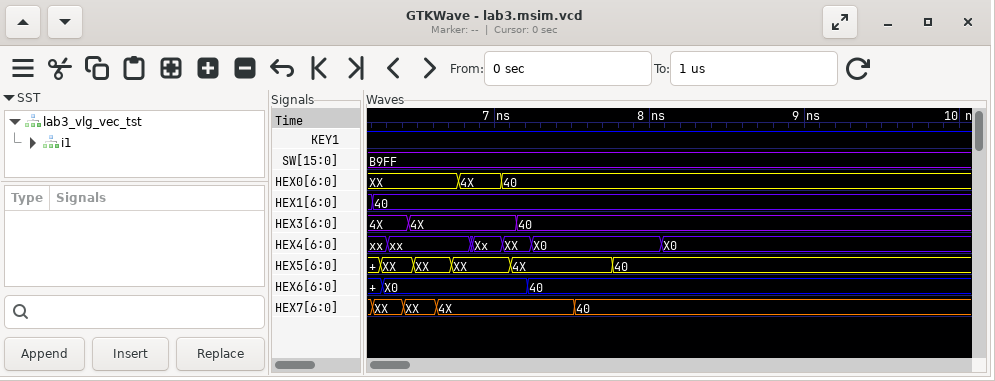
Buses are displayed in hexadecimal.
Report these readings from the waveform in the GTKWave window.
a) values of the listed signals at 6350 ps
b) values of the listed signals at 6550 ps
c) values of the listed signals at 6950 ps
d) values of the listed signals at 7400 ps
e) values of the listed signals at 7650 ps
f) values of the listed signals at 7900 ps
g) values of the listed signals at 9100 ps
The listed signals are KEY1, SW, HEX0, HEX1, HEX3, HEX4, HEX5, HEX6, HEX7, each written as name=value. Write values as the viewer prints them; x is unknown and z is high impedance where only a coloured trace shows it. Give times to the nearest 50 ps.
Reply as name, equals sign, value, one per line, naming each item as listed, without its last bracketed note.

values of the listed signals at 6350 ps = KEY1=1, SW=B9FF, HEX0=XX, HEX1=40, HEX3=4X, HEX4=xx, HEX5=XX, HEX6=X0, HEX7=XX
values of the listed signals at 6550 ps = KEY1=1, SW=B9FF, HEX0=XX, HEX1=40, HEX3=4X, HEX4=xx, HEX5=XX, HEX6=X0, HEX7=XX
values of the listed signals at 6950 ps = KEY1=1, SW=B9FF, HEX0=4X, HEX1=40, HEX3=4X, HEX4=Xx, HEX5=XX, HEX6=X0, HEX7=4X
values of the listed signals at 7400 ps = KEY1=1, SW=B9FF, HEX0=40, HEX1=40, HEX3=40, HEX4=X0, HEX5=4X, HEX6=40, HEX7=4X
values of the listed signals at 7650 ps = KEY1=1, SW=B9FF, HEX0=40, HEX1=40, HEX3=40, HEX4=X0, HEX5=4X, HEX6=40, HEX7=40
values of the listed signals at 7900 ps = KEY1=1, SW=B9FF, HEX0=40, HEX1=40, HEX3=40, HEX4=X0, HEX5=40, HEX6=40, HEX7=40
values of the listed signals at 9100 ps = KEY1=1, SW=B9FF, HEX0=40, HEX1=40, HEX3=40, HEX4=X0, HEX5=40, HEX6=40, HEX7=40
